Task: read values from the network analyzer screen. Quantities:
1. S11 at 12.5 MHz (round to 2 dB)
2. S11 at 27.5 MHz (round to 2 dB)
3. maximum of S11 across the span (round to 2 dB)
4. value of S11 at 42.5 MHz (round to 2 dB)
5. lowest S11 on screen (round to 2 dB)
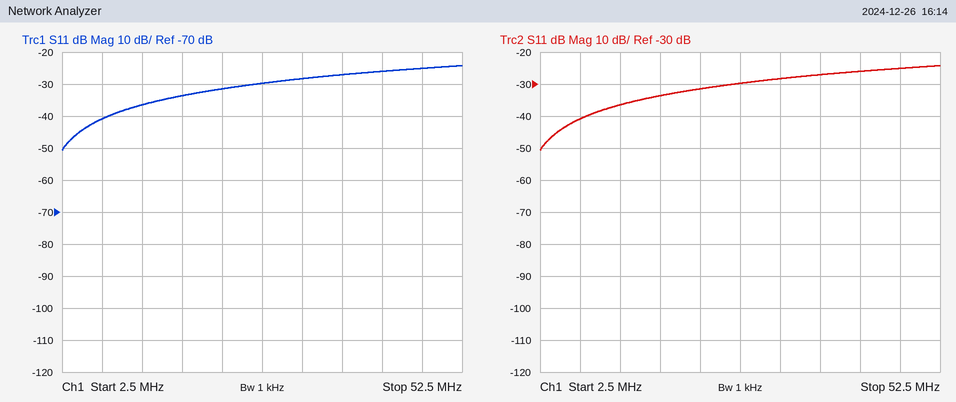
-36 dB
-30 dB
-24 dB
-26 dB
-50 dB
